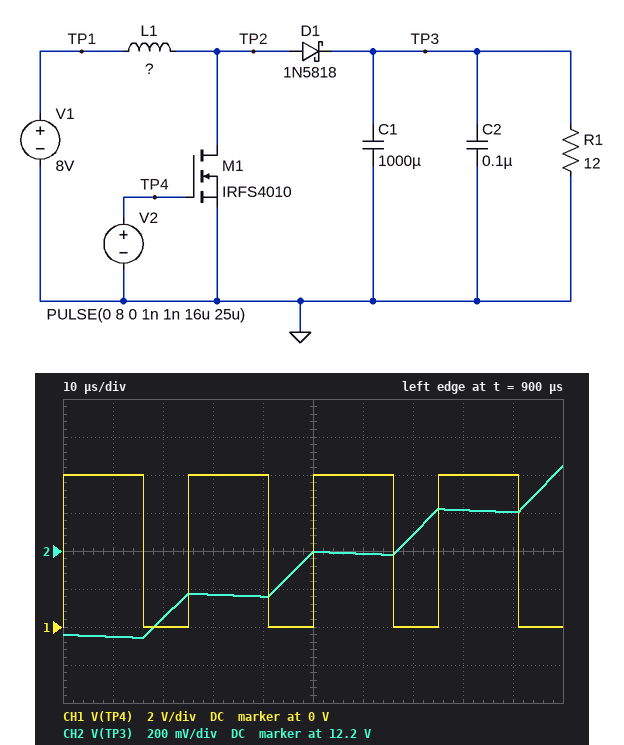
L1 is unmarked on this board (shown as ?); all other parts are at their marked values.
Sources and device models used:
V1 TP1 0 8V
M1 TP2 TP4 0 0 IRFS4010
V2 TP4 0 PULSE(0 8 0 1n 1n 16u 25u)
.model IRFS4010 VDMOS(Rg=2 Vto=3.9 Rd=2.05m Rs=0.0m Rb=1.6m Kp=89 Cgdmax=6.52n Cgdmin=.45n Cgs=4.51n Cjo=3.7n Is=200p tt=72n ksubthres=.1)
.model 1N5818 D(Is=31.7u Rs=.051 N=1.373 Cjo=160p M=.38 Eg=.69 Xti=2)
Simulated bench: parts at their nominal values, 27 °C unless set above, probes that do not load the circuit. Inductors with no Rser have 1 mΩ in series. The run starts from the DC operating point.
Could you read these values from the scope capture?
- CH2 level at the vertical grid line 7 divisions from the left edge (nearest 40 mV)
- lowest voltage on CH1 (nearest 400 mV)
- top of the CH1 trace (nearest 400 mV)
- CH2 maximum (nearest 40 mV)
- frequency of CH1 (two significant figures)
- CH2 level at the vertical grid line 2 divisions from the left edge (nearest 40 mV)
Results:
12.28 V
0 V
8.0 V
12.64 V
40 kHz
11.84 V
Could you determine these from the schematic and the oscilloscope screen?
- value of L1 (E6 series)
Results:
150 µH
